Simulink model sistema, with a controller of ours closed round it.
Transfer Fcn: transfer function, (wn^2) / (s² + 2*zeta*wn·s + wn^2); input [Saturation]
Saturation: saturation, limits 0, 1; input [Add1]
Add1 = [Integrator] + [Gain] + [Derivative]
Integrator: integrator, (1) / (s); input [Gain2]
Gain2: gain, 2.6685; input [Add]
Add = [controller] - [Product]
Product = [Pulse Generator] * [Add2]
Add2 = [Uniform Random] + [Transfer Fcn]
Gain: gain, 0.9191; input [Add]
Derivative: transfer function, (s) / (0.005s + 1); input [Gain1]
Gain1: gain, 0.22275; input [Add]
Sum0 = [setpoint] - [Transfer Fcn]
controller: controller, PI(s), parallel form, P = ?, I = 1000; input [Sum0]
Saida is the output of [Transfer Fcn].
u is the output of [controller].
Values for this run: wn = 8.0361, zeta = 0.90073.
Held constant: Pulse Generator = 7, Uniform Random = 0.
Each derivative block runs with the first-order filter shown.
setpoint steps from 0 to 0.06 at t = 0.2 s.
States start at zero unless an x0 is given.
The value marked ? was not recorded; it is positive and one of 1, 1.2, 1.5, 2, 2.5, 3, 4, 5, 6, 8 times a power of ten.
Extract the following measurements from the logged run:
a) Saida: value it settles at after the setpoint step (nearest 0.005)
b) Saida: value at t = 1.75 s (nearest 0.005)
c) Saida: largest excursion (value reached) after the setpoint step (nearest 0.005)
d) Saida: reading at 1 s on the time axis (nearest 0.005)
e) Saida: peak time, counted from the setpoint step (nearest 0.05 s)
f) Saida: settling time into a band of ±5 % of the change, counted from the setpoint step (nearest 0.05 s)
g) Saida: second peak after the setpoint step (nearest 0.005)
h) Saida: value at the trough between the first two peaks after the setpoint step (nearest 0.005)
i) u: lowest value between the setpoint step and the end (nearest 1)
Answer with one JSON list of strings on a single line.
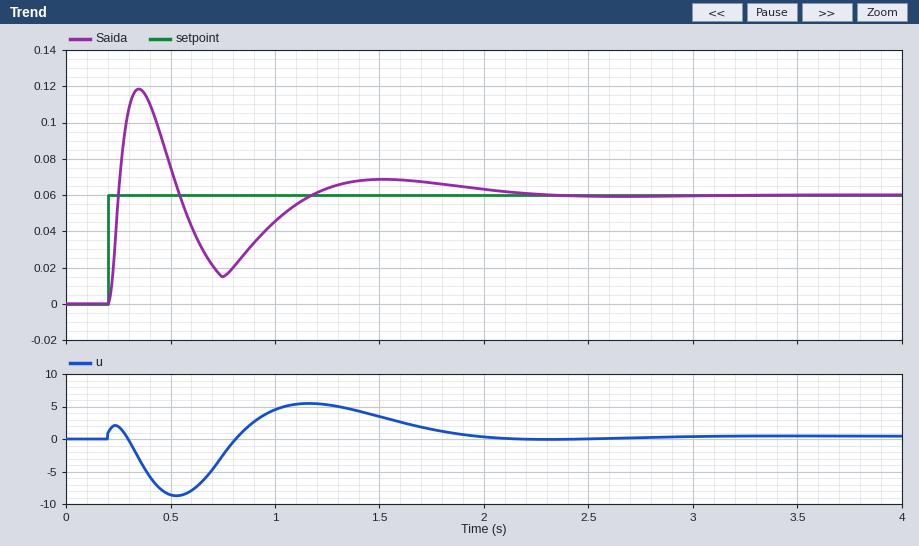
["0.060", "0.065", "0.120", "0.045", "0.15 s", "1.80 s", "0.070", "0.015", "-9"]
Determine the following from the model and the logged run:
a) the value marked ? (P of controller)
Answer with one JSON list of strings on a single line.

["15"]
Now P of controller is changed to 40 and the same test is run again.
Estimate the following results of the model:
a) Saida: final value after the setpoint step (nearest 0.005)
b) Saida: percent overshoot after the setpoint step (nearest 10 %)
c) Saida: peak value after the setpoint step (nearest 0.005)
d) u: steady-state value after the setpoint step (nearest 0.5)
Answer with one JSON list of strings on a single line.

["0.060", "40 %", "0.085", "0.5"]
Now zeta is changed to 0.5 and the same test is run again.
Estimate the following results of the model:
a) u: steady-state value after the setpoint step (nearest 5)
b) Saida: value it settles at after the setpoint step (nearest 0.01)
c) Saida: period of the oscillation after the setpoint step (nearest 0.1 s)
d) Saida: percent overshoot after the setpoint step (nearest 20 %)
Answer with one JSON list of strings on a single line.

["0", "0.06", "1.2 s", "160 %"]
